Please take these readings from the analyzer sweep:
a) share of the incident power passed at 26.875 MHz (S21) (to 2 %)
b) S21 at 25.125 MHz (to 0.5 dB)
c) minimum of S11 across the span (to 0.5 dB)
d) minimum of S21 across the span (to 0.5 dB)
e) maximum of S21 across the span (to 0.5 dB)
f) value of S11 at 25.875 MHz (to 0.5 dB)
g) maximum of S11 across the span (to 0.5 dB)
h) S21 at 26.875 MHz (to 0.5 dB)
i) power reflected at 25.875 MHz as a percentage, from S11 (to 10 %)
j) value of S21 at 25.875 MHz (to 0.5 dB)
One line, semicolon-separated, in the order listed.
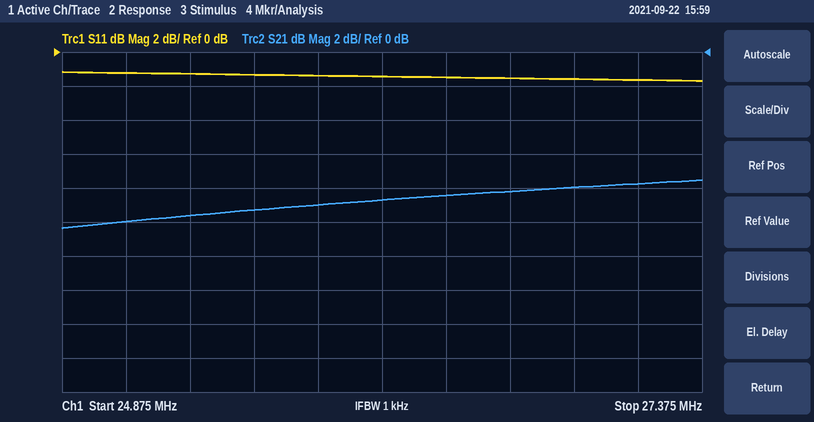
16 %; -10.0 dB; -1.5 dB; -10.5 dB; -7.5 dB; -1.5 dB; -1.0 dB; -8.0 dB; 70 %; -9.0 dB
